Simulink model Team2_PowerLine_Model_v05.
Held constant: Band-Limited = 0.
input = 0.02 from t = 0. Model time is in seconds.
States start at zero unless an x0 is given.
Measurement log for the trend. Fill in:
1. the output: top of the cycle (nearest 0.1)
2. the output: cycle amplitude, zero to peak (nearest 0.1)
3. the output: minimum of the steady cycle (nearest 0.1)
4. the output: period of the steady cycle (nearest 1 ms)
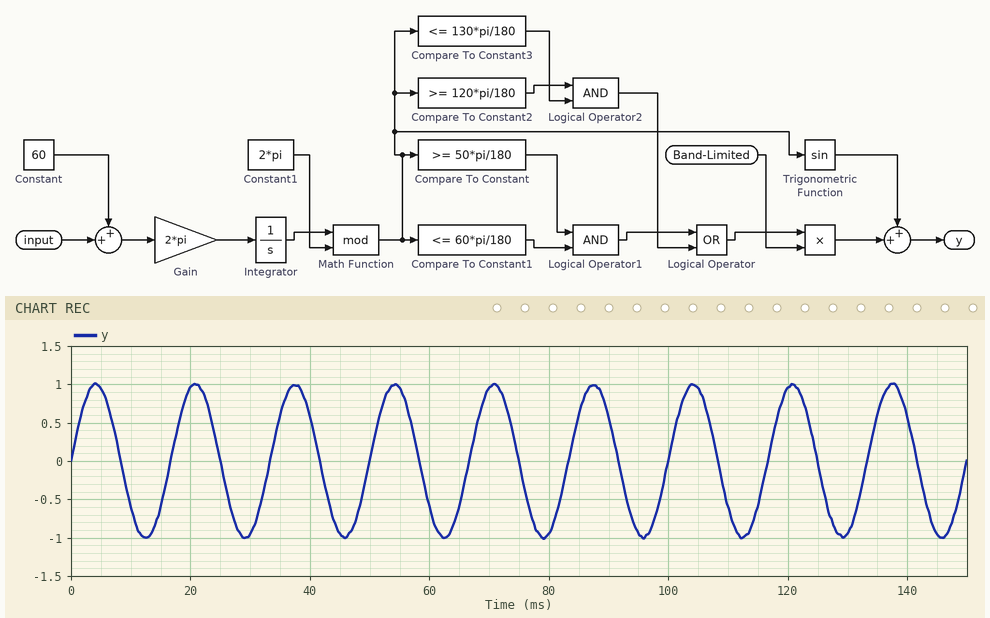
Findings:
1.0
1.0
-1.0
17 ms
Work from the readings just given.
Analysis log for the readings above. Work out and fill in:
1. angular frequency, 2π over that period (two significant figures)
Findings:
0.37 rad/ms
